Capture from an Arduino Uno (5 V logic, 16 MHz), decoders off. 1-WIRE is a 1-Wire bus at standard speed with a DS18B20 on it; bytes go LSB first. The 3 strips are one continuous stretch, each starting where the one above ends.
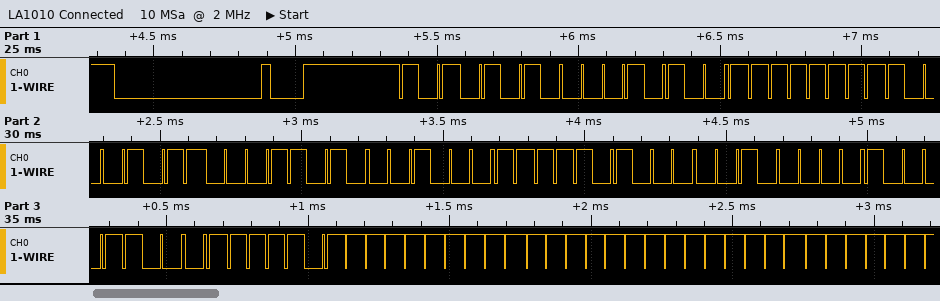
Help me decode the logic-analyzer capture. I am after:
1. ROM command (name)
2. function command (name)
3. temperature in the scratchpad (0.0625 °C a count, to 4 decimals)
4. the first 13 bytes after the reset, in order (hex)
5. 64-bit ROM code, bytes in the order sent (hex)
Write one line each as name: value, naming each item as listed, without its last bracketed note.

ROM command: Match ROM
function command: Read Scratchpad
temperature in the scratchpad: -0.0625 °C
the first 13 bytes after the reset, in order: 55 28 FF D1 58 C4 17 04 31 BE FF FF FF
64-bit ROM code, bytes in the order sent: 28 FF D1 58 C4 17 04 31
